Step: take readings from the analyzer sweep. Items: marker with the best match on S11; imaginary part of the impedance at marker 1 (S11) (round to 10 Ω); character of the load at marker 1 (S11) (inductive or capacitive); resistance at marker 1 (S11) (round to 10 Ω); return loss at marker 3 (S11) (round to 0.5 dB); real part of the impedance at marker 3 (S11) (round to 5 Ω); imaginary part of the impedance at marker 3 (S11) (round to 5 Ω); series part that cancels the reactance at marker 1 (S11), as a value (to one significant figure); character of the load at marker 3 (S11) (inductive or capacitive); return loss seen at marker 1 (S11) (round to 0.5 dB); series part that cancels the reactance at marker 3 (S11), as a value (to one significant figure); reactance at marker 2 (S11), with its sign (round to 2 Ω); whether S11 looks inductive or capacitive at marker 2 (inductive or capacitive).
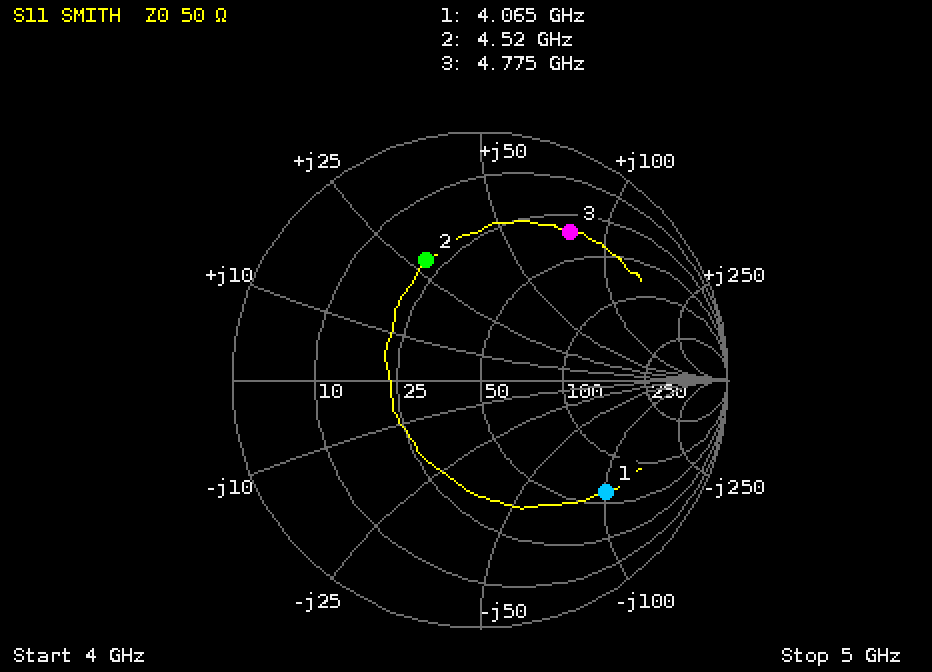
marker 2
-100 Ω
capacitive
60 Ω
3.0 dB
35 Ω
+80 Ω
4 nH
inductive
3.5 dB
400 fF
+28 Ω
inductive
